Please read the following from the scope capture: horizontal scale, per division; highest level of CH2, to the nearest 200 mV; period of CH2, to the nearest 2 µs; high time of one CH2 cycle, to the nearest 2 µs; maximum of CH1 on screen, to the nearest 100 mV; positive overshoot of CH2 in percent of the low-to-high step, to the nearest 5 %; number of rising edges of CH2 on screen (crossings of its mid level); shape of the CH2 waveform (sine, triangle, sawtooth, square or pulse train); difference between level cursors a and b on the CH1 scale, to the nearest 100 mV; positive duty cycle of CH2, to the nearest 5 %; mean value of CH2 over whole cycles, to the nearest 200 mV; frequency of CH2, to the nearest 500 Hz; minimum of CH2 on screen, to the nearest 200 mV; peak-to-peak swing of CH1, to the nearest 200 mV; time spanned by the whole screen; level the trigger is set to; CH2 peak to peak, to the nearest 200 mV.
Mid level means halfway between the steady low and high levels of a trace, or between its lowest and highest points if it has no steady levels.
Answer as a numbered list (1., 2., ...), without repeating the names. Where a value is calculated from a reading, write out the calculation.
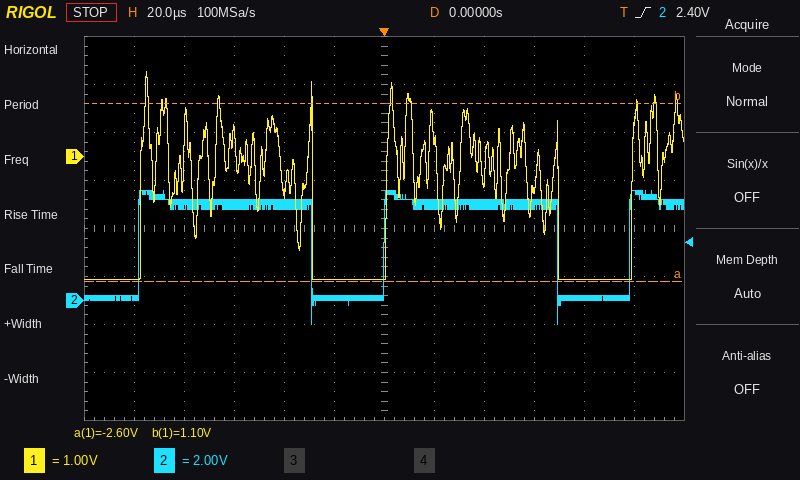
1. 20 µs
2. 4.6 V
3. 98 µs
4. 70 µs
5. 1.8 V
6. 15 %
7. 3
8. pulse train
9. 3.7 V
10. 70 µs / 98 µs ≈ 71.4 %, so 70 % to the nearest 5 %
11. -1.0 V + 0.7 × (4.6 V − (-1.0 V)) ≈ 2.92 V, so 3.0 V to the nearest 200 mV
12. 1 / 98 µs ≈ 10.2 kHz, so 10.0 kHz to the nearest 500 Hz
13. -1.0 V
14. 4.4 V
15. 240 µs
16. 2.40 V
17. 4.6 V − (-1.0 V) = 5.6 V
